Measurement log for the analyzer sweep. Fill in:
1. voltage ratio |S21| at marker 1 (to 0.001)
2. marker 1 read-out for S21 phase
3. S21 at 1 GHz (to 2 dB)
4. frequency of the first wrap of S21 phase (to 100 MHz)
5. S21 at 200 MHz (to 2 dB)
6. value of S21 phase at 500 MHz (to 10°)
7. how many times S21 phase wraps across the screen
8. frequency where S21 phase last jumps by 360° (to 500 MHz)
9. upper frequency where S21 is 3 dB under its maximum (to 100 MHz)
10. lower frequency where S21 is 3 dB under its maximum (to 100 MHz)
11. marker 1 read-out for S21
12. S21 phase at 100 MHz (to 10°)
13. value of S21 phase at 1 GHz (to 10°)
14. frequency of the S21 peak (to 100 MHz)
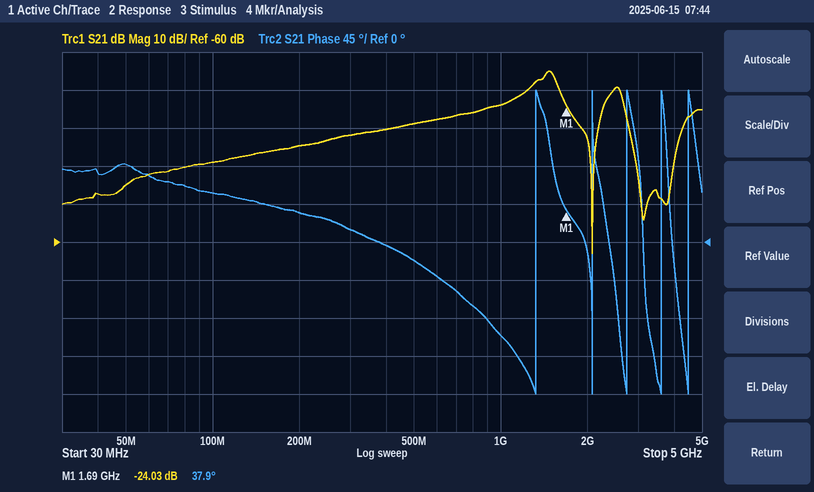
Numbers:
0.063
37.9°
-24 dB
1.3 GHz
-34 dB
-20°
5
4.5 GHz
1.6 GHz
1.3 GHz
-24.03 dB
60°
-110°
1.5 GHz
